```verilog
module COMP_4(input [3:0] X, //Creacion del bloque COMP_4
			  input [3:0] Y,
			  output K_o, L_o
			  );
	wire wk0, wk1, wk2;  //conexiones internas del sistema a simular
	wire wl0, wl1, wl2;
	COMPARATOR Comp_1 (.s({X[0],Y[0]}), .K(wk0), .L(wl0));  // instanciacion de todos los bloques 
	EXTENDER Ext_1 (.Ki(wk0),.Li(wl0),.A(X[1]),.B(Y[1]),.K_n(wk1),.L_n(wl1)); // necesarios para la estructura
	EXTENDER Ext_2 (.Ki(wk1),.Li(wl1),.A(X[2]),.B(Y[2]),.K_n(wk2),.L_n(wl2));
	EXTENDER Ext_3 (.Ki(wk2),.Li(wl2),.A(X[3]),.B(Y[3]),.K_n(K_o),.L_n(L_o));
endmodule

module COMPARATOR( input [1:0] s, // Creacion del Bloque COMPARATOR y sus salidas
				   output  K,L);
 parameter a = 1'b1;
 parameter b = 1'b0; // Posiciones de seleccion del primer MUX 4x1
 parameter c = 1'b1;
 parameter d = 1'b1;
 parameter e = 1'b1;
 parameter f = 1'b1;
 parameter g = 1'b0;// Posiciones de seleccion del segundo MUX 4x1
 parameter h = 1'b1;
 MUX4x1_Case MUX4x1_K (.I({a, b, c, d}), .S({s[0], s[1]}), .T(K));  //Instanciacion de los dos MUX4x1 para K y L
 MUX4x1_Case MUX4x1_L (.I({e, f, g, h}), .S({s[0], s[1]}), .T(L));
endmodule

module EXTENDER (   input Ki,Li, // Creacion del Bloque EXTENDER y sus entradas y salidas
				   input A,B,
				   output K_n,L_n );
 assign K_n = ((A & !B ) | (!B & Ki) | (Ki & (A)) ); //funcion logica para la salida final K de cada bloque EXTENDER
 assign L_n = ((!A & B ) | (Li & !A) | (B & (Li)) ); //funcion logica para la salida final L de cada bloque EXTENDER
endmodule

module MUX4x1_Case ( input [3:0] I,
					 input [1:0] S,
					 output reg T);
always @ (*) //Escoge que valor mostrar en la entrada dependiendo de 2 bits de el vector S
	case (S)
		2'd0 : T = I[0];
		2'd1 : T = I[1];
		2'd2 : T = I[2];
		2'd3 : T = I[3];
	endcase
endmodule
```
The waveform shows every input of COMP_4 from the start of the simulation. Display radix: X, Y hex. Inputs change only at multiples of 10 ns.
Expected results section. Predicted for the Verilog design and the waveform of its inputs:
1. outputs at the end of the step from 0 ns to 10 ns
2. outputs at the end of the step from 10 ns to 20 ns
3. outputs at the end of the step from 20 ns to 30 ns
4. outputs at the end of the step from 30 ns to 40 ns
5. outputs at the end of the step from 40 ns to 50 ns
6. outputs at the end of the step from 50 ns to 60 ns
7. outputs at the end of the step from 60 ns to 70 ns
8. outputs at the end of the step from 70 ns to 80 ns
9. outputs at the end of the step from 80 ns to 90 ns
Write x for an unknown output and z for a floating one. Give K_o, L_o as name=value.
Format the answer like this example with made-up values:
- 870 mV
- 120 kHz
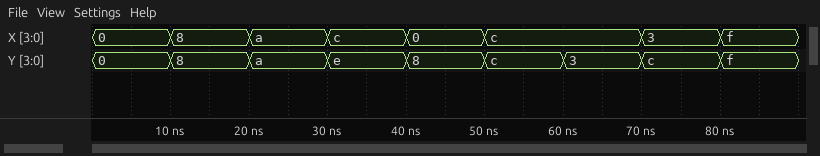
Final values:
- K_o=1, L_o=1
- K_o=1, L_o=1
- K_o=1, L_o=1
- K_o=0, L_o=1
- K_o=0, L_o=1
- K_o=1, L_o=1
- K_o=1, L_o=0
- K_o=0, L_o=1
- K_o=1, L_o=1
